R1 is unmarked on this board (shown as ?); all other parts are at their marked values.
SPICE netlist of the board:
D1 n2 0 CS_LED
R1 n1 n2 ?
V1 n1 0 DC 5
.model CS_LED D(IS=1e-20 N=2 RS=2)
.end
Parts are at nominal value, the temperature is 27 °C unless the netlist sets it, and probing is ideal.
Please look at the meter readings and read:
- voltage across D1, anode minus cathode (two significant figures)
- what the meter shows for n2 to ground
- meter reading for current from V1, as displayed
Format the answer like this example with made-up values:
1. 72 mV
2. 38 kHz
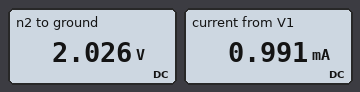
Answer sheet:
1. 2.0 V
2. 2.026 V
3. 0.991 mA
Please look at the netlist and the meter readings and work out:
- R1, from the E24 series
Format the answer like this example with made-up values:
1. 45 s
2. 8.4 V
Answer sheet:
1. 3 kΩ
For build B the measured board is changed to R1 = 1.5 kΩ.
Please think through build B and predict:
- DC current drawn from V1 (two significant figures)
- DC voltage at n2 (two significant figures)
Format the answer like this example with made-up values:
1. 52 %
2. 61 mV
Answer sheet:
1. 2.0 mA
2. 2.1 V
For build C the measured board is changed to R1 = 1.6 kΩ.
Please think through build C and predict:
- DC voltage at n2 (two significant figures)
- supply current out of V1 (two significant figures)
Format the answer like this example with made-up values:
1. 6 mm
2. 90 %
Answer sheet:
1. 2.1 V
2. 1.8 mA
